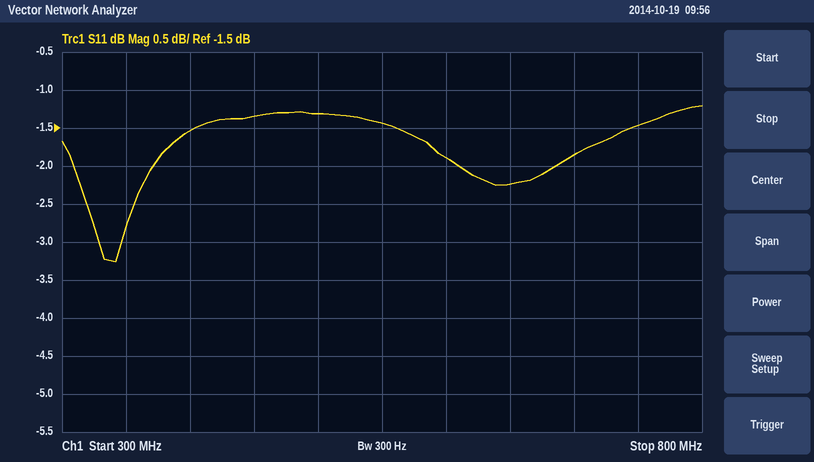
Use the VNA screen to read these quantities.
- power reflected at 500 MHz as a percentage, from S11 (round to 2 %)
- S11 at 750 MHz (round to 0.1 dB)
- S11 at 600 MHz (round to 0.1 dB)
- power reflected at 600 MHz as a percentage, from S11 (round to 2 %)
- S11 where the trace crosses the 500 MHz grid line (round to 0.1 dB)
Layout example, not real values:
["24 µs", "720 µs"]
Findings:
["74 %", "-1.5 dB", "-1.9 dB", "64 %", "-1.3 dB"]
